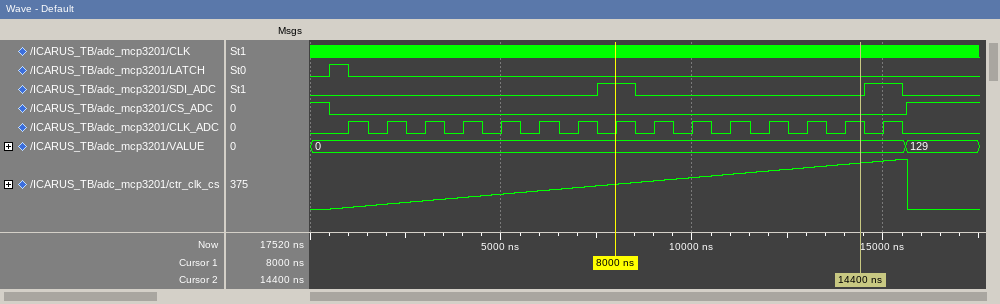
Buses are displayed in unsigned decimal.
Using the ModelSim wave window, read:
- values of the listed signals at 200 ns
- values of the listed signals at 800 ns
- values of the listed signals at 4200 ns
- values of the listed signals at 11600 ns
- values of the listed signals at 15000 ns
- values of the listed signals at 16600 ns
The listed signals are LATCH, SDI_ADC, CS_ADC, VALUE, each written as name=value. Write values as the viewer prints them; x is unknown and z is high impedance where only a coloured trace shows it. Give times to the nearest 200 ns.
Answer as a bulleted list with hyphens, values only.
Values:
- LATCH=0, SDI_ADC=0, CS_ADC=1, VALUE=0
- LATCH=1, SDI_ADC=0, CS_ADC=0, VALUE=0
- LATCH=0, SDI_ADC=0, CS_ADC=0, VALUE=0
- LATCH=0, SDI_ADC=0, CS_ADC=0, VALUE=0
- LATCH=0, SDI_ADC=1, CS_ADC=0, VALUE=0
- LATCH=0, SDI_ADC=0, CS_ADC=1, VALUE=129
